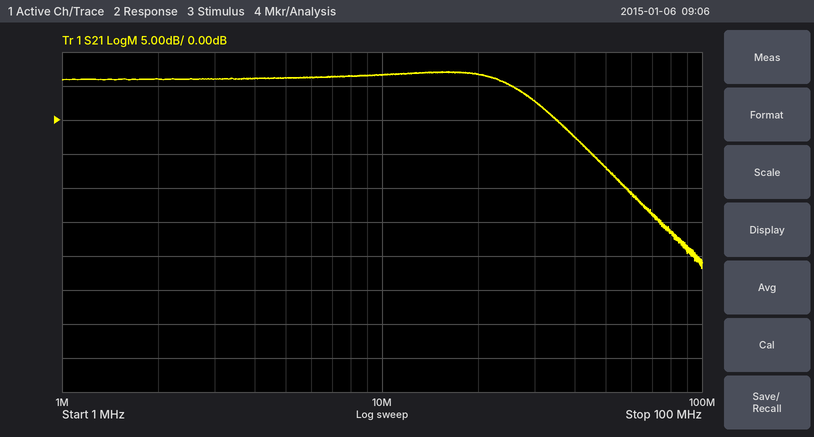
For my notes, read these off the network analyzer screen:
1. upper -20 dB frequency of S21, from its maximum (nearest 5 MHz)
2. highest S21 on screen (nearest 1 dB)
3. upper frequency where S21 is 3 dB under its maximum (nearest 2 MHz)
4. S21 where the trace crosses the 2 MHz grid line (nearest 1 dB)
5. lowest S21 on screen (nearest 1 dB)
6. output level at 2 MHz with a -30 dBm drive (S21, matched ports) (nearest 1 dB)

65 MHz
7 dB
28 MHz
6 dB
-22 dB
-24 dBm
